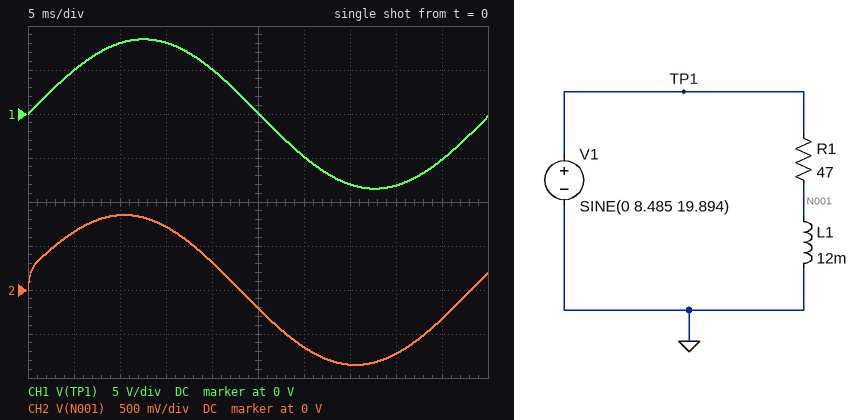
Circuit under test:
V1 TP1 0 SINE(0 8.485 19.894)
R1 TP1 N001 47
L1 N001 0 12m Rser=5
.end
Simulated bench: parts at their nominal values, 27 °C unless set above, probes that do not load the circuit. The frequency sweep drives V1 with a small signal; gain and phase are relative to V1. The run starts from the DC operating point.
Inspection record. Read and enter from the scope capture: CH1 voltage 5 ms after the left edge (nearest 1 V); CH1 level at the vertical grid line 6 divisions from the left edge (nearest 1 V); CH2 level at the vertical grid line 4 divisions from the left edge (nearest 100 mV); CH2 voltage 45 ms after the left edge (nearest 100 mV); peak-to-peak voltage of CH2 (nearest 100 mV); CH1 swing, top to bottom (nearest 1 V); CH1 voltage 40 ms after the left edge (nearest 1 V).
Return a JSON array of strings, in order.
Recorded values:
["5 V", "-5 V", "300 mV", "-300 mV", "1.7 V", "17 V", "-8 V"]
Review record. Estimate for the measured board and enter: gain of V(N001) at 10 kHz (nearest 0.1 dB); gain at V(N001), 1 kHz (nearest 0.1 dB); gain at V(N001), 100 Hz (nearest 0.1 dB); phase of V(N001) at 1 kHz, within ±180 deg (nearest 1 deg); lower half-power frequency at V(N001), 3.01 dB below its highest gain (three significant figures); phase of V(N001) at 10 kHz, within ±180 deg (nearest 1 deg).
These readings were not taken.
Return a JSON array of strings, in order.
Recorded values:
["0 dB", "-1.7 dB", "-15.3 dB", "31 deg", "683 Hz", "4 deg"]
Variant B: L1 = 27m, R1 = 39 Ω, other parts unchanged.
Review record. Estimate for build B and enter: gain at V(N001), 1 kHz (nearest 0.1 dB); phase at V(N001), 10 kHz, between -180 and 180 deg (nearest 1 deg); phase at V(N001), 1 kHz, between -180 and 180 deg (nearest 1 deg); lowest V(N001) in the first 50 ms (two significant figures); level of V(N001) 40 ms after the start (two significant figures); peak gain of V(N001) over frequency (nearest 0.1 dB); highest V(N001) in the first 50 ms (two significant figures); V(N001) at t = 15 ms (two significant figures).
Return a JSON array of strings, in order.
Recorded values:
["-0.3 dB", "1 deg", "13 deg", "-1.2 V", "-800 mV", "0 dB", "1.2 V", "790 mV"]
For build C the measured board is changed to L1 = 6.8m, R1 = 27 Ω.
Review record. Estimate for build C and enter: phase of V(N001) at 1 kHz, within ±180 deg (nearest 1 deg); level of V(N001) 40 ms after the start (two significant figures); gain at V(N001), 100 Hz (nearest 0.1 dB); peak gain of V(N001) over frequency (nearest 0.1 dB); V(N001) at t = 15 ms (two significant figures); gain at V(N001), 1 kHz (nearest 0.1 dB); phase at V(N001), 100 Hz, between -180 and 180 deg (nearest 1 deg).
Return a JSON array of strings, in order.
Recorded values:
["30 deg", "-1.2 V", "-13.8 dB", "0 dB", "1.2 V", "-1.9 dB", "33 deg"]
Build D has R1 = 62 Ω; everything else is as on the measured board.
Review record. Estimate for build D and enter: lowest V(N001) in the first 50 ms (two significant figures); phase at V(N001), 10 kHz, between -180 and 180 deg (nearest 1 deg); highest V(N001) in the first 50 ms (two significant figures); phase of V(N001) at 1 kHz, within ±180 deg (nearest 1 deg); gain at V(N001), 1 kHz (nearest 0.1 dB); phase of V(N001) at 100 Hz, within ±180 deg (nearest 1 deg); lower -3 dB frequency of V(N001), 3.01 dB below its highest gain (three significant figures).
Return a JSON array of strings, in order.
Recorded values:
["-660 mV", "5 deg", "660 mV", "38 deg", "-2.5 dB", "50 deg", "884 Hz"]
